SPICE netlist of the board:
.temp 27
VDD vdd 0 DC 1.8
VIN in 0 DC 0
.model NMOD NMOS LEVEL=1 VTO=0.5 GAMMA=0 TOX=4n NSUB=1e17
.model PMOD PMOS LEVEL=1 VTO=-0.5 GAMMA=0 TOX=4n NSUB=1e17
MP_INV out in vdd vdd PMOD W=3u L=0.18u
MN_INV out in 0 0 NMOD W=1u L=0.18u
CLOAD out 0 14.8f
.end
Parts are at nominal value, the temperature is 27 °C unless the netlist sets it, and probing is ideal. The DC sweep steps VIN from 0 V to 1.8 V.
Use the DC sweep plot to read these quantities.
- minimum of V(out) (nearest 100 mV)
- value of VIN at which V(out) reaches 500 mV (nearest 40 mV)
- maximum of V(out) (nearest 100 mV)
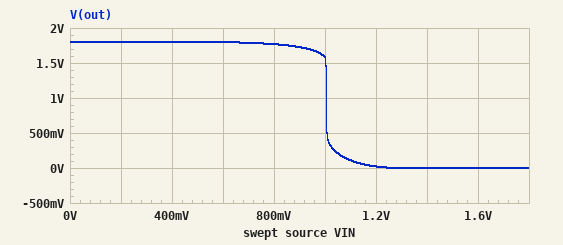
0 V
1.00 V
1.8 V
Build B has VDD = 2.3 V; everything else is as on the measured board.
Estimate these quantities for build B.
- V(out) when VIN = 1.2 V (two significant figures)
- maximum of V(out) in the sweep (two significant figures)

2.1 V
2.3 V
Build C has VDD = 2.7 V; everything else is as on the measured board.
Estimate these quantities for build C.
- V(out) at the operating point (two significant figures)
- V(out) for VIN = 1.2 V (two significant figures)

2.7 V
2.6 V
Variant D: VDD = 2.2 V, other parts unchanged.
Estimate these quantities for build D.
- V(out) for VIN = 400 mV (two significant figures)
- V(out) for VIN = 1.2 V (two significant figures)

2.2 V
2.0 V
